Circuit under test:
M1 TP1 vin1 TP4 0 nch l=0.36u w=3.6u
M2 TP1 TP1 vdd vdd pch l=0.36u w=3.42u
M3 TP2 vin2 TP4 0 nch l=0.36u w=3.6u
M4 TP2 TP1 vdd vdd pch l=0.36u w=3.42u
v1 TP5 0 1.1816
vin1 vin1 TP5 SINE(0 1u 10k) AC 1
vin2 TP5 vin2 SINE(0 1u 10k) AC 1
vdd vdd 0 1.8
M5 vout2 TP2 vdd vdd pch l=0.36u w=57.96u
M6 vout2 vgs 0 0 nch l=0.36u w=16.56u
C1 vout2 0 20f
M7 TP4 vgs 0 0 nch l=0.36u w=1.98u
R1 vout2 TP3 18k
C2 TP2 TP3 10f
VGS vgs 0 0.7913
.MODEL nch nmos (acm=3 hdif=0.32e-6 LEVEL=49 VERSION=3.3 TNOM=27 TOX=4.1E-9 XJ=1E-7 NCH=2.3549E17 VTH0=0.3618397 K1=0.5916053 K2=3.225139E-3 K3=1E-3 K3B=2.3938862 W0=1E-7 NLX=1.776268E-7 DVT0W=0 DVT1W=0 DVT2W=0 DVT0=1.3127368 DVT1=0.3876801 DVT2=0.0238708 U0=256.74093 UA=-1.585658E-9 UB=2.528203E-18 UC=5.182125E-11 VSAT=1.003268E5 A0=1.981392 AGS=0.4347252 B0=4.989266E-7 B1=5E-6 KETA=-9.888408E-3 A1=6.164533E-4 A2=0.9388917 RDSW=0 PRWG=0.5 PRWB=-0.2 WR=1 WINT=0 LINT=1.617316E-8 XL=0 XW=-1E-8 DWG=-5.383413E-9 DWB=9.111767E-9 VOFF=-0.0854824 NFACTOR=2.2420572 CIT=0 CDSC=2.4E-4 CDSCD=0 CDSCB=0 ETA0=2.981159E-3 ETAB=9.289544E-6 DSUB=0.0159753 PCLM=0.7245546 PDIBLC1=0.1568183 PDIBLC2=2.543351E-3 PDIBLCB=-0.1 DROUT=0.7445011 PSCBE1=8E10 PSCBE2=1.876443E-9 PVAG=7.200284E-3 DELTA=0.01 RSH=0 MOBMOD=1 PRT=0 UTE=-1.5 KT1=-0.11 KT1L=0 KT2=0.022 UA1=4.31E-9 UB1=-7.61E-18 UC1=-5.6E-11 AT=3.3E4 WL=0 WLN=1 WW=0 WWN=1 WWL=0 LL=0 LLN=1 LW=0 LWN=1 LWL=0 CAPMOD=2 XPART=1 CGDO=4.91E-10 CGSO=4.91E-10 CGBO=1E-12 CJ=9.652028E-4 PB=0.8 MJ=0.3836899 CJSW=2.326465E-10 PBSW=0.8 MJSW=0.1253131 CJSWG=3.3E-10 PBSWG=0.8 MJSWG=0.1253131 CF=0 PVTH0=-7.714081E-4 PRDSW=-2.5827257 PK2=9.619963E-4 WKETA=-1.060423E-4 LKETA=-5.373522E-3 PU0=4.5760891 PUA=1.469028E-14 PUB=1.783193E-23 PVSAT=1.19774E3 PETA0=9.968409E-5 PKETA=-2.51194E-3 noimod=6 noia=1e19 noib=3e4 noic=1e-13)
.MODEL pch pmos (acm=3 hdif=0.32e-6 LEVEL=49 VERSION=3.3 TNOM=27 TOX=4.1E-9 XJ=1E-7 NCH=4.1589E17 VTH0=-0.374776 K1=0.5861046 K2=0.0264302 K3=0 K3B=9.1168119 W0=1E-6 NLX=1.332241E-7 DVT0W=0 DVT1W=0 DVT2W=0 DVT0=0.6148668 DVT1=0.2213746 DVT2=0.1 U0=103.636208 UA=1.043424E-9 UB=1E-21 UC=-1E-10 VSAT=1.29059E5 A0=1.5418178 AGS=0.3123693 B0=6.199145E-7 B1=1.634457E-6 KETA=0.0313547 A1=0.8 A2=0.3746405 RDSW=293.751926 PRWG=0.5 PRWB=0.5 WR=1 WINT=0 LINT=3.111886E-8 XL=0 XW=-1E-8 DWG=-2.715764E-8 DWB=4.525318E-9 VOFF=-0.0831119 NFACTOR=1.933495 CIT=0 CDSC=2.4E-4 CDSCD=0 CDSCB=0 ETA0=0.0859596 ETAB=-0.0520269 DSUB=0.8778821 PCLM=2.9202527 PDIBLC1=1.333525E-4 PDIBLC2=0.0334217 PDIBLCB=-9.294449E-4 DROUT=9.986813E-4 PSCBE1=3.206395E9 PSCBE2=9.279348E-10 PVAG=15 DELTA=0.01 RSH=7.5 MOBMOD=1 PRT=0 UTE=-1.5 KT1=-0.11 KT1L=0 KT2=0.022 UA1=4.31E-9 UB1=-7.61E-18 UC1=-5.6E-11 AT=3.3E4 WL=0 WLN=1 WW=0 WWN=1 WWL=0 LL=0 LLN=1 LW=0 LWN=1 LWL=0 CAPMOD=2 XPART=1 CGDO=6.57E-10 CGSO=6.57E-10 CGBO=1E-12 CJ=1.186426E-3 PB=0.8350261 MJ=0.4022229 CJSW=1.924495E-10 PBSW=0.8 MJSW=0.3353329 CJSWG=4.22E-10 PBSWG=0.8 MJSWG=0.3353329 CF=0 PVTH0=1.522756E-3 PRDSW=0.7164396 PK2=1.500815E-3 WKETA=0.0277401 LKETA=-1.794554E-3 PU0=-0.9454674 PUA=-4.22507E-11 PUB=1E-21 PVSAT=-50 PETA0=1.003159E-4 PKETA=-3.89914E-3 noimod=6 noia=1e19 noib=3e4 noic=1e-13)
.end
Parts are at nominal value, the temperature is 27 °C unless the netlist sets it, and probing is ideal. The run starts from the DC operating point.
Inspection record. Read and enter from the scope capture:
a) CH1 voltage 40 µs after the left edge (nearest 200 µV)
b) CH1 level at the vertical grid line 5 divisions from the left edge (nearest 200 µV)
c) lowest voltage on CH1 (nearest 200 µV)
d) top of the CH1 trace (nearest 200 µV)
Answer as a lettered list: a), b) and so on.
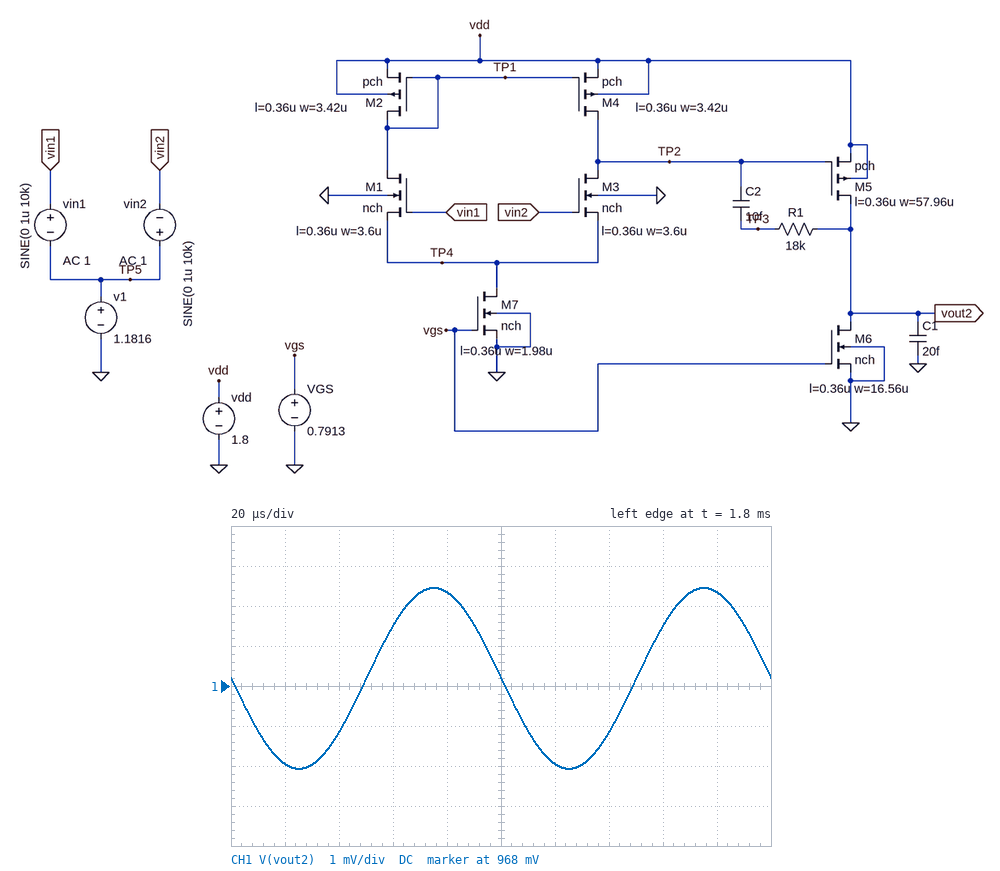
a) 966.8 mV
b) 968.2 mV
c) 966.0 mV
d) 970.4 mV
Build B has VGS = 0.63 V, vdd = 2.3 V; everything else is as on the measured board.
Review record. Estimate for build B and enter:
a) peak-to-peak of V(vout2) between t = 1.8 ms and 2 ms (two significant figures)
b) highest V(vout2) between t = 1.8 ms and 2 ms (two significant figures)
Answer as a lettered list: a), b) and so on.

a) 7.2 mV
b) 1.3 V
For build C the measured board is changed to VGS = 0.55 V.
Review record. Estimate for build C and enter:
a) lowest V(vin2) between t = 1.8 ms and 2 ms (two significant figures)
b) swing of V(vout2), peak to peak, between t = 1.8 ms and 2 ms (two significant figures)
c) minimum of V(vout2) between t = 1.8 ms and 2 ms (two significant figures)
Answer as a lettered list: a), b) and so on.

a) 1.2 V
b) 7.0 mV
c) 1.0 V
